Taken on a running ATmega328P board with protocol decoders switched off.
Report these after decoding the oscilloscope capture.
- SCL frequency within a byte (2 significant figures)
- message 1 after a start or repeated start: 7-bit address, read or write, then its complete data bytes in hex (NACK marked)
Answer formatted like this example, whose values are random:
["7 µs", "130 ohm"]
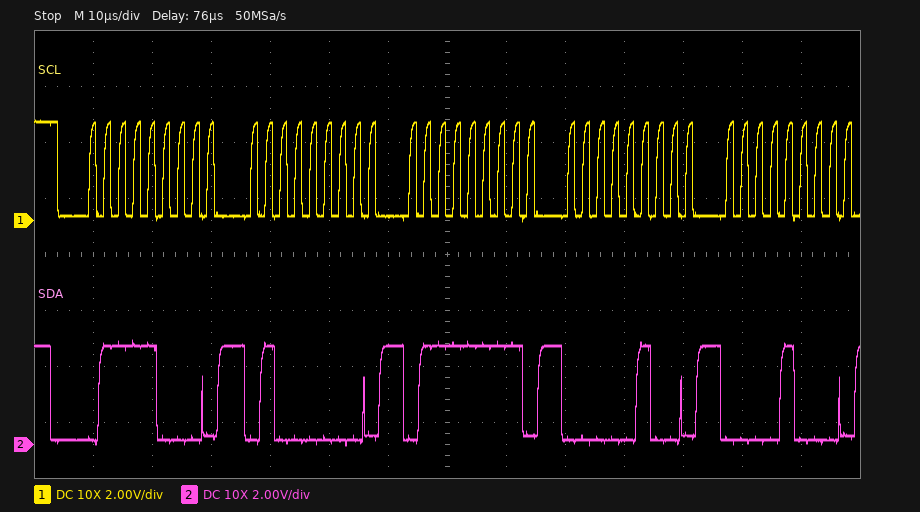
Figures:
["400 kHz", "0x3C write: 40 7F 04 08"]
